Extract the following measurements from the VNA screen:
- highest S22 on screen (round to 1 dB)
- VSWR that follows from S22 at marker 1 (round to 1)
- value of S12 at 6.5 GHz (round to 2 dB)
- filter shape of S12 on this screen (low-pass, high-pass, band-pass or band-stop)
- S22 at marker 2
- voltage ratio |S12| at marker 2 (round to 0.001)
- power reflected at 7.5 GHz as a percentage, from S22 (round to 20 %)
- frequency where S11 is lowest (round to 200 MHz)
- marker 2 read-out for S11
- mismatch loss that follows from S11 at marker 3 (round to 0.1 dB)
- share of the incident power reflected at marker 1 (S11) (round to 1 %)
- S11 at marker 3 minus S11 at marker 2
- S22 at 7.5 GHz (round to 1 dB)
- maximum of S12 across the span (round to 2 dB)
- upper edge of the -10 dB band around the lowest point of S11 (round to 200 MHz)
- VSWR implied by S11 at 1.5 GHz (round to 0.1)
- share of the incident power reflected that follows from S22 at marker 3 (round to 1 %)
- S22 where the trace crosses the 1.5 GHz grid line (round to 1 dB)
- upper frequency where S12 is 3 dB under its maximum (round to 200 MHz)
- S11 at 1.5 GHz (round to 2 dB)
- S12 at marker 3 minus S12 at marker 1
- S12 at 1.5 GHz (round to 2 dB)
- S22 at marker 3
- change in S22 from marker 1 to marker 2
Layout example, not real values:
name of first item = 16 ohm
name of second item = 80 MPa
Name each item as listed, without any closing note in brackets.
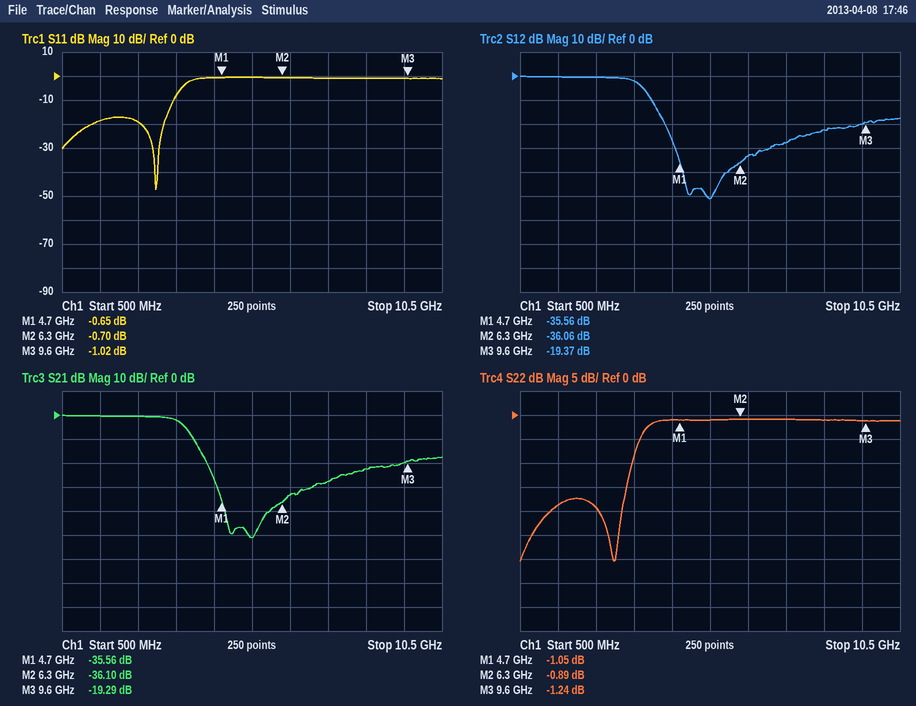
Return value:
highest S22 on screen = -1 dB
VSWR that follows from S22 at marker 1 = 17
value of S12 at 6.5 GHz = -34 dB
filter shape of S12 on this screen = low-pass
S22 at marker 2 = -0.89 dB
voltage ratio |S12| at marker 2 = 0.016
power reflected at 7.5 GHz as a percentage, from S22 = 80 %
frequency where S11 is lowest = 3.0 GHz
marker 2 read-out for S11 = -0.70 dB
mismatch loss that follows from S11 at marker 3 = 6.8 dB
share of the incident power reflected at marker 1 (S11) = 86 %
S11 at marker 3 minus S11 at marker 2 = -0.32 dB
S22 at 7.5 GHz = -1 dB
maximum of S12 across the span = 0 dB
upper edge of the -10 dB band around the lowest point of S11 = 3.4 GHz
VSWR implied by S11 at 1.5 GHz = 1.3
share of the incident power reflected that follows from S22 at marker 3 = 75 %
S22 where the trace crosses the 1.5 GHz grid line = -19 dB
upper frequency where S12 is 3 dB under its maximum = 3.6 GHz
S11 at 1.5 GHz = -18 dB
S12 at marker 3 minus S12 at marker 1 = 16.19 dB
S12 at 1.5 GHz = 0 dB
S22 at marker 3 = -1.24 dB
change in S22 from marker 1 to marker 2 = 0.16 dB
